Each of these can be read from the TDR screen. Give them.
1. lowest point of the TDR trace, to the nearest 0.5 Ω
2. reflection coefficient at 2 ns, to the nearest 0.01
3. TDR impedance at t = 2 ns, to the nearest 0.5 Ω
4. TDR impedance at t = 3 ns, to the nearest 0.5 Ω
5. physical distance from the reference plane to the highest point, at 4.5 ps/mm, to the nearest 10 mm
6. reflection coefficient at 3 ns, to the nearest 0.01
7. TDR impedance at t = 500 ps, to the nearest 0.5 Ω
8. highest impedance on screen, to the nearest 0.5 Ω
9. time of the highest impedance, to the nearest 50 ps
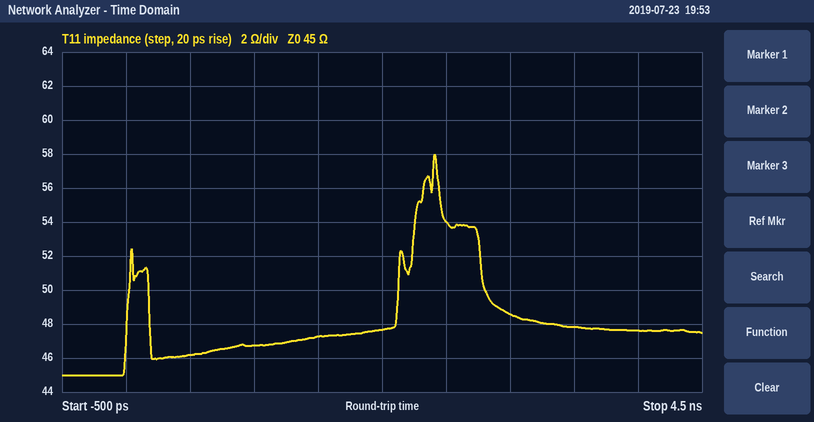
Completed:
45.0 Ω
+0.03
47.5 Ω
48.5 Ω
270 mm
+0.04
46.0 Ω
58.0 Ω
2.40 ns
